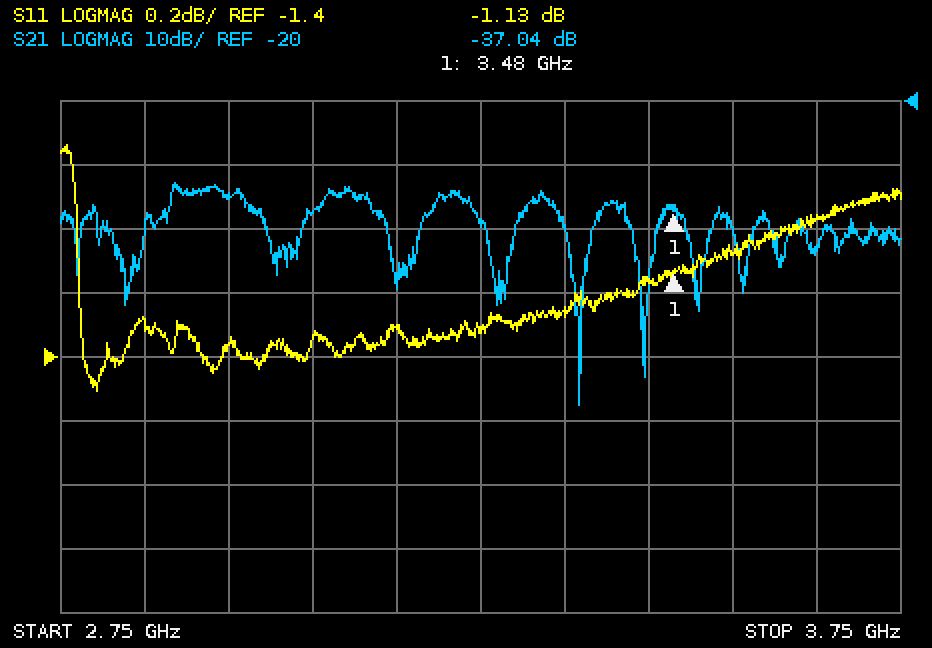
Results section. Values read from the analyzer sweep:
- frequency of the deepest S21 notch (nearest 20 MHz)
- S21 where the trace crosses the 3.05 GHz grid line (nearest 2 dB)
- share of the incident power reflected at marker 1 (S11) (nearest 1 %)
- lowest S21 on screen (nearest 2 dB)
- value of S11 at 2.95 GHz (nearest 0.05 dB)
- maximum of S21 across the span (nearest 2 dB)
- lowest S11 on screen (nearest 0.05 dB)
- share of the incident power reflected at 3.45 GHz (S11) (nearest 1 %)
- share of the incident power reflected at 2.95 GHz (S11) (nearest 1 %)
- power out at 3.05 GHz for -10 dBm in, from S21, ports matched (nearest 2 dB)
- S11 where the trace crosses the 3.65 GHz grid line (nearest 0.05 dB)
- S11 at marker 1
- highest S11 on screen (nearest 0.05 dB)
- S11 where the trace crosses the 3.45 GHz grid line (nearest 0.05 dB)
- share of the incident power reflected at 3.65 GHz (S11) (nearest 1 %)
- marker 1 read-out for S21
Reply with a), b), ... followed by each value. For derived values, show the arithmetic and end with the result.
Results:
a) 3.36 GHz
b) -38 dB
c) 10^(-1.13/10) ≈ 77 %
d) -68 dB
e) -1.35 dB
f) -32 dB
g) -1.50 dB
h) 10^(-1.15/10) ≈ 77 %
i) 10^(-1.35/10) ≈ 73 %
j) -10 dBm + (-38 dB) = -48 dBm
k) -0.95 dB
l) -1.13 dB
m) -0.75 dB
n) -1.15 dB
o) 10^(-0.95/10) ≈ 80 %
p) -37.04 dB
